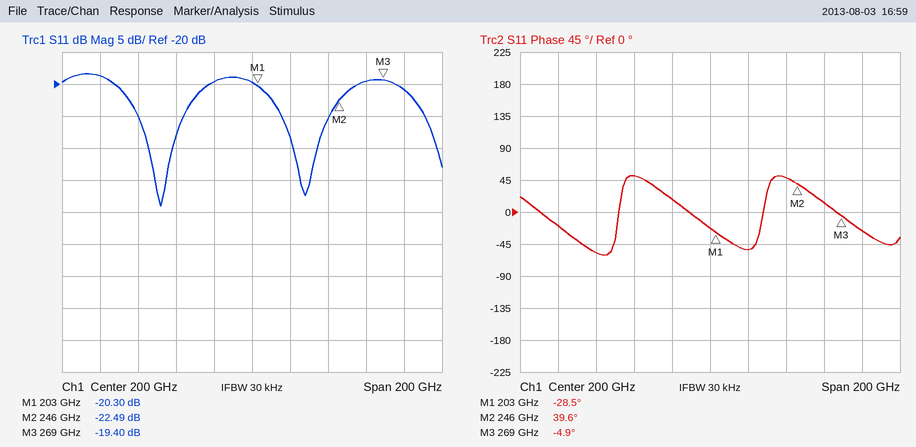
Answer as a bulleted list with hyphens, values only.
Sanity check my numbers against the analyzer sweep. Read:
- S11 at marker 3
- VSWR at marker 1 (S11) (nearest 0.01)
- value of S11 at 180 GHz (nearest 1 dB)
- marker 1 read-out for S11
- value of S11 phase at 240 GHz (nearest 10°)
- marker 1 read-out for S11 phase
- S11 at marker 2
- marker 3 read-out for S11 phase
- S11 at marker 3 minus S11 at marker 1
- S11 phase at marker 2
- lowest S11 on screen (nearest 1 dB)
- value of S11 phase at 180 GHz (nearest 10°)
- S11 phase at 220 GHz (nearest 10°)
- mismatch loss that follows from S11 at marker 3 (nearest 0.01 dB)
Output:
- -19.40 dB
- 1.21
- -20 dB
- -20.30 dB
- 50°
- -28.5°
- -22.49 dB
- -4.9°
- 0.90 dB
- 39.6°
- -39 dB
- 20°
- -50°
- 0.05 dB
